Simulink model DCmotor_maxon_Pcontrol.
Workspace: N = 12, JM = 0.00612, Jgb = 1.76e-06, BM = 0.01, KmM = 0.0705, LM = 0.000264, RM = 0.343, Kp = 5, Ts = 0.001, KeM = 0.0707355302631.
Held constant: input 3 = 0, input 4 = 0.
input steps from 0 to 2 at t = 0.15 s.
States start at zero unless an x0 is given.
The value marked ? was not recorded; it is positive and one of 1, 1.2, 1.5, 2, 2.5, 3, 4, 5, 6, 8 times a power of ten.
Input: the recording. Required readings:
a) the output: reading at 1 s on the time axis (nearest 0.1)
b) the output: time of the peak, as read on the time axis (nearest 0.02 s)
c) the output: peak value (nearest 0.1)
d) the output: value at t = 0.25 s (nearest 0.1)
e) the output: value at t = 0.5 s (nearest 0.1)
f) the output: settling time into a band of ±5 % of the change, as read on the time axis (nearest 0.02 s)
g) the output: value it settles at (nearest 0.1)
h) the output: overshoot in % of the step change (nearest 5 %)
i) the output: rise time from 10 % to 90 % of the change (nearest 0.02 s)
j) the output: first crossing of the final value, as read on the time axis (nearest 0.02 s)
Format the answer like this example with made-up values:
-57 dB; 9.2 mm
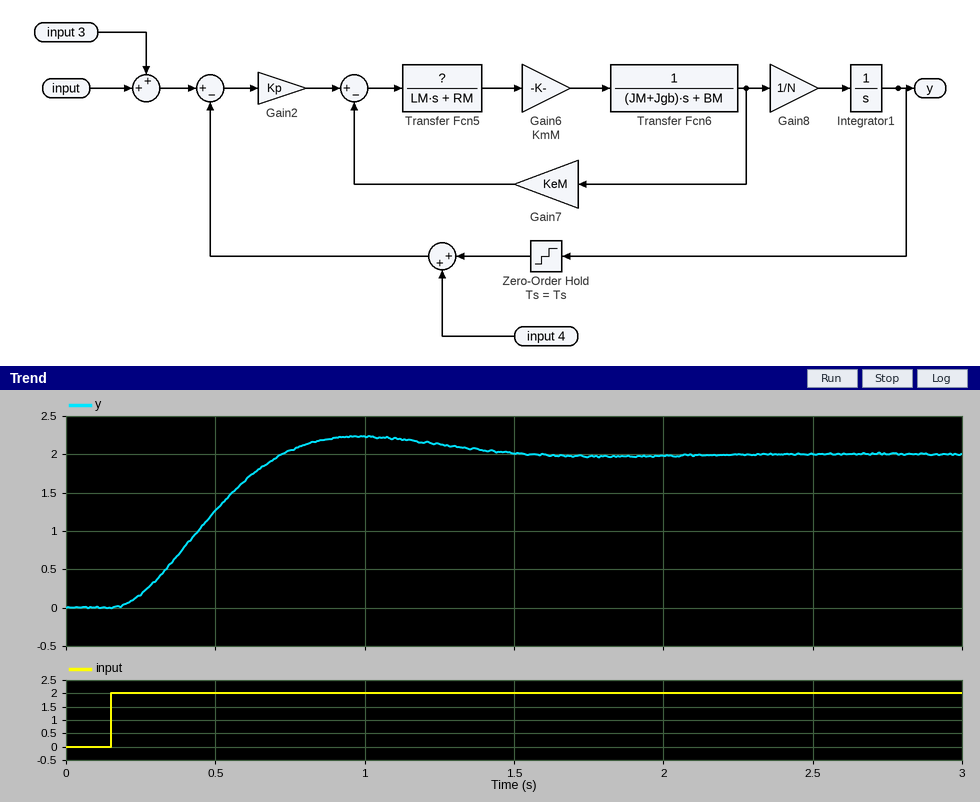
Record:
2.2; 0.98 s; 2.2; 0.2; 1.3; 1.30 s; 2.0; 10 %; 0.38 s; 0.72 s
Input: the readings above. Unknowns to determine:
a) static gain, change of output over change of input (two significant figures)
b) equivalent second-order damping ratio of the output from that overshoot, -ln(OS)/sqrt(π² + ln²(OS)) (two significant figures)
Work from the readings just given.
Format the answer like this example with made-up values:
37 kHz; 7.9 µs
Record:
1.0; 0.59
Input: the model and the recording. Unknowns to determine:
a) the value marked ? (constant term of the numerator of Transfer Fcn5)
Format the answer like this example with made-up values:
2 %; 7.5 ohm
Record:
1.5
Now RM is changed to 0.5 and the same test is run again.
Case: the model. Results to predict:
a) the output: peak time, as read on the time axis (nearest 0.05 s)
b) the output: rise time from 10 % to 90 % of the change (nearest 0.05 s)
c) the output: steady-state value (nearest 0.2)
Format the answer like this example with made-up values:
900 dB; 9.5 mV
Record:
1.15 s; 0.45 s; 2.0
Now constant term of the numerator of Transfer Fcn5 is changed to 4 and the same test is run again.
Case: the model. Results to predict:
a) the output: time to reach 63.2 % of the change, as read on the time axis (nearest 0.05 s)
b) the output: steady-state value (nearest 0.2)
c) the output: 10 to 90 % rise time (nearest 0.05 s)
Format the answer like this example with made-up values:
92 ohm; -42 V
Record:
0.40 s; 2.0; 0.30 s
